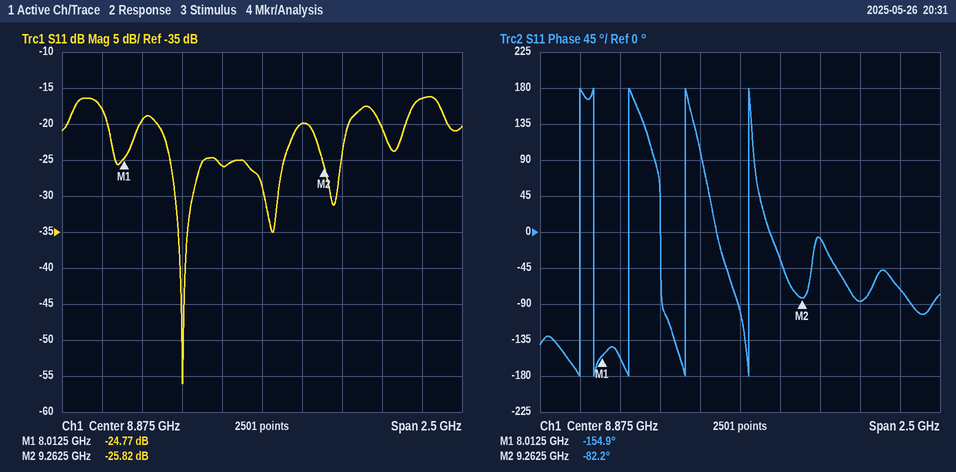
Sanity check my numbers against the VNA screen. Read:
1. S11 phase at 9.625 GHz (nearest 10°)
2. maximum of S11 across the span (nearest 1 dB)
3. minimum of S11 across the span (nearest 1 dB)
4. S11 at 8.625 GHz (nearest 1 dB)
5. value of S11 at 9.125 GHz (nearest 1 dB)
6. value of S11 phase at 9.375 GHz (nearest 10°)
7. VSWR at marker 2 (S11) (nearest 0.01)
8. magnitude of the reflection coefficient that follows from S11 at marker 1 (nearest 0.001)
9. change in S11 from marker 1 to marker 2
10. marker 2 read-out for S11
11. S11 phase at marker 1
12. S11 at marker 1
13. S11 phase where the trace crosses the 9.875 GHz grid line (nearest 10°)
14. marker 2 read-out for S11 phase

-90°
-16 dB
-56 dB
-26 dB
-20 dB
-10°
1.11
0.058
-1.05 dB
-25.82 dB
-154.9°
-24.77 dB
-70°
-82.2°
